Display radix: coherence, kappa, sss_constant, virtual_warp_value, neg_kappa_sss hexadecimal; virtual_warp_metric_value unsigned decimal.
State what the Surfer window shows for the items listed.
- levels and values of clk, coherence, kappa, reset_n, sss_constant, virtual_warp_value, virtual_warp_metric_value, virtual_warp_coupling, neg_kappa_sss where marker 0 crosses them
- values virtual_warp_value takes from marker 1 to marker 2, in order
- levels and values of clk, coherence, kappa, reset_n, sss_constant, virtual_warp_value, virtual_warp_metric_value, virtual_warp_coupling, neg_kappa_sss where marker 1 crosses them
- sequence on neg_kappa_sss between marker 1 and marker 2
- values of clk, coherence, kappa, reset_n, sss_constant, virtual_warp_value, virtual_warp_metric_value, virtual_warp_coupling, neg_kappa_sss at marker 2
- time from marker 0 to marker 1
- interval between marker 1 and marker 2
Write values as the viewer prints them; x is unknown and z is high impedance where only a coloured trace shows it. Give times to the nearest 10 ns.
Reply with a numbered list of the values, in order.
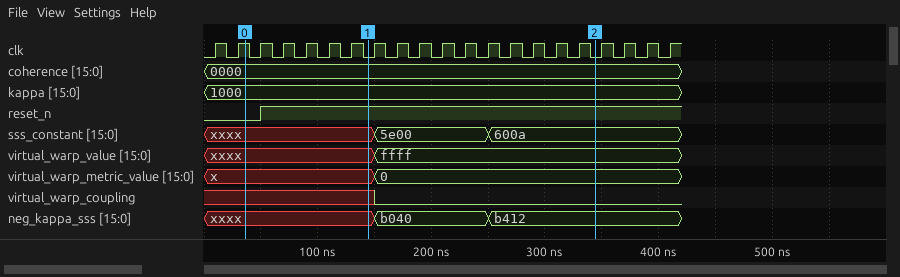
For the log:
1. clk=1, coherence=0000, kappa=1000, reset_n=0, sss_constant=xxxx, virtual_warp_value=xxxx, virtual_warp_metric_value=x, virtual_warp_coupling=x, neg_kappa_sss=xxxx
2. xxxx, ffff
3. clk=0, coherence=0000, kappa=1000, reset_n=1, sss_constant=xxxx, virtual_warp_value=xxxx, virtual_warp_metric_value=x, virtual_warp_coupling=x, neg_kappa_sss=xxxx
4. xxxx, b040, b412
5. clk=0, coherence=0000, kappa=1000, reset_n=1, sss_constant=600a, virtual_warp_value=ffff, virtual_warp_metric_value=0, virtual_warp_coupling=0, neg_kappa_sss=b412
6. 110 ns
7. 200 ns
